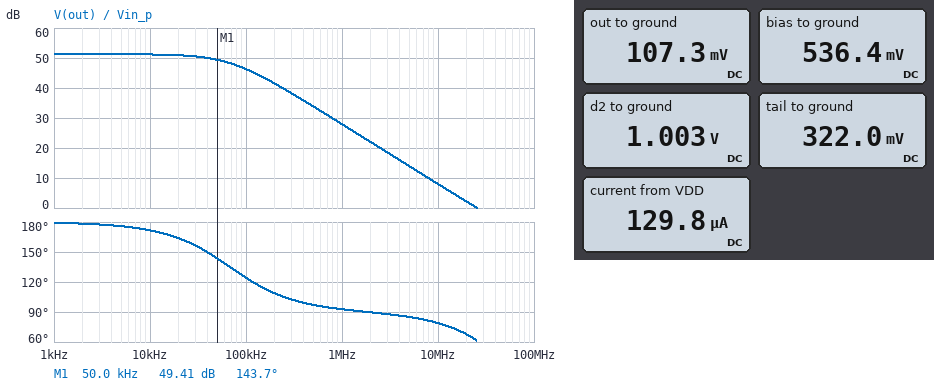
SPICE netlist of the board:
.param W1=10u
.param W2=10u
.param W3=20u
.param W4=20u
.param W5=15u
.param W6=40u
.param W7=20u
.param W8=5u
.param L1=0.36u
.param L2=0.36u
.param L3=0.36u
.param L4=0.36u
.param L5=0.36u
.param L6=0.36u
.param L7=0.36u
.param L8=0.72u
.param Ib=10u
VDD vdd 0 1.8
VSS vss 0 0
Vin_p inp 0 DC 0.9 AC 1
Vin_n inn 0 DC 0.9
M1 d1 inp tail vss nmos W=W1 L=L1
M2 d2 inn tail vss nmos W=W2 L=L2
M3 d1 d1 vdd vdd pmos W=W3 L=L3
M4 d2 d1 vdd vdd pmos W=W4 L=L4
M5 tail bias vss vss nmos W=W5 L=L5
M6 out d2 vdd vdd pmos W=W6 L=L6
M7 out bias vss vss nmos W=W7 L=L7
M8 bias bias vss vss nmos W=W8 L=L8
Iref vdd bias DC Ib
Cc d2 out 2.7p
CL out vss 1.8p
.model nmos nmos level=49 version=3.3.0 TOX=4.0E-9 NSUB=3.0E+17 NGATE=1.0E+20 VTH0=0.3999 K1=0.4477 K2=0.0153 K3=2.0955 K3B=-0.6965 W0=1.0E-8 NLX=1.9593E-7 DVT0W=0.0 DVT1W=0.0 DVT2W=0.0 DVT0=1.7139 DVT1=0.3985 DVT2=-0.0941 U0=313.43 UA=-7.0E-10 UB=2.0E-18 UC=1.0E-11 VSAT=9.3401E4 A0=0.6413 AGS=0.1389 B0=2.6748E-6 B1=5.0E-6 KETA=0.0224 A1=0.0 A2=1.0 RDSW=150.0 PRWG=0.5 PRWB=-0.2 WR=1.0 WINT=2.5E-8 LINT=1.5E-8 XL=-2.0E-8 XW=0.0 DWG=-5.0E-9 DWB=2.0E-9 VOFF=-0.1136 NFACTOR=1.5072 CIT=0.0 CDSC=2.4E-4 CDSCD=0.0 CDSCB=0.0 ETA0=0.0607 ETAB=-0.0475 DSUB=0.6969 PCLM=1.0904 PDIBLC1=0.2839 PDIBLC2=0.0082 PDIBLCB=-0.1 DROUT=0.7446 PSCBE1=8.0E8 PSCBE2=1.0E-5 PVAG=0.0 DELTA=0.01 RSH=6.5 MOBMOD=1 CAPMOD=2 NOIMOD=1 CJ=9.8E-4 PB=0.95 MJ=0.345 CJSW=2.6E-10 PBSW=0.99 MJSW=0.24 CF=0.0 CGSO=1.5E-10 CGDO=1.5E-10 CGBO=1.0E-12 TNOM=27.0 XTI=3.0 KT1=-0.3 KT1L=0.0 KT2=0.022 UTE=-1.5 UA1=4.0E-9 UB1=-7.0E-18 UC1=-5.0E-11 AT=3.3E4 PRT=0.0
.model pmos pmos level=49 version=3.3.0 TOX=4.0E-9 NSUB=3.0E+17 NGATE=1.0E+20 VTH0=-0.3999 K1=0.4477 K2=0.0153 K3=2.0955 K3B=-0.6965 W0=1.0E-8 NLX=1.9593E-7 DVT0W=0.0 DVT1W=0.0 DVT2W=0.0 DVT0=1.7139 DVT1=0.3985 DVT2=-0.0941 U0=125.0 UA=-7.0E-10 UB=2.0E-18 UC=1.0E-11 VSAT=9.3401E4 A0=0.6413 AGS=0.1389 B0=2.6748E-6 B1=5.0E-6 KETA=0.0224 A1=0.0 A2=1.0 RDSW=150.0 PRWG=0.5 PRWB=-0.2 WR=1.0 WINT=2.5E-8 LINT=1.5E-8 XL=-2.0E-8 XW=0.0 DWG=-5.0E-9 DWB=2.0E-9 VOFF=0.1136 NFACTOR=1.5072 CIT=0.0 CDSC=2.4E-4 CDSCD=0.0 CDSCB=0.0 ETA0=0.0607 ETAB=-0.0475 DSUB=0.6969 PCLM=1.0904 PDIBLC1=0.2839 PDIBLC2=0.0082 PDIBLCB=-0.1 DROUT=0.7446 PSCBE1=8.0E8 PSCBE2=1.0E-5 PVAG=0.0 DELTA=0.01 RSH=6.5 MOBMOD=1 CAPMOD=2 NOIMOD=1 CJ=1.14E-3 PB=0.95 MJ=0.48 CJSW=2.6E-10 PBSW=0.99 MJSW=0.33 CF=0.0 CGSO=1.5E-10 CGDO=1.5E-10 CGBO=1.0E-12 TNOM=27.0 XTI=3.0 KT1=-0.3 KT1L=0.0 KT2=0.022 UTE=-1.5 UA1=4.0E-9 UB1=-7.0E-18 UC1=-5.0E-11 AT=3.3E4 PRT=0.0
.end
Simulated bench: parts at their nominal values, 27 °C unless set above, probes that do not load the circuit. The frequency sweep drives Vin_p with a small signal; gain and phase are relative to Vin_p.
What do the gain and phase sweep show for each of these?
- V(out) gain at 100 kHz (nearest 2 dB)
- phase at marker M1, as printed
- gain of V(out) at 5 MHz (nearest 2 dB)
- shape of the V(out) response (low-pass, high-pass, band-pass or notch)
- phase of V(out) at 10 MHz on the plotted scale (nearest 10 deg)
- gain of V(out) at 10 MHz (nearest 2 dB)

46 dB
143.7 deg
14 dB
low-pass
80 deg
8 dB
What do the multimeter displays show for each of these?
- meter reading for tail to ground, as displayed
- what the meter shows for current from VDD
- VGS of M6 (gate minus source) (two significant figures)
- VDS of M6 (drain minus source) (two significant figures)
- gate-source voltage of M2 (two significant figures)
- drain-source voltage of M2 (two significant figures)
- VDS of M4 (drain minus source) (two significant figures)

322.0 mV
129.8 µA
-800 mV
-1.7 V
580 mV
680 mV
-800 mV
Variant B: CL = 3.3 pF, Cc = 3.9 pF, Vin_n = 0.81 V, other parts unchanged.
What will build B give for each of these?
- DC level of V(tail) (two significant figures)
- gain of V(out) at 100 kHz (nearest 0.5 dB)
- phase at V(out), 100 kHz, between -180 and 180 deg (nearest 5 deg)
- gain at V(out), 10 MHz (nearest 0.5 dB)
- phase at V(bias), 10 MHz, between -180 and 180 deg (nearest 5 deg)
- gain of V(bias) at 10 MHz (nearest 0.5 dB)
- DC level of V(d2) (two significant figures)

300 mV
-62.0 dB
90 deg
-24.0 dB
110 deg
-60.0 dB
1.8 V
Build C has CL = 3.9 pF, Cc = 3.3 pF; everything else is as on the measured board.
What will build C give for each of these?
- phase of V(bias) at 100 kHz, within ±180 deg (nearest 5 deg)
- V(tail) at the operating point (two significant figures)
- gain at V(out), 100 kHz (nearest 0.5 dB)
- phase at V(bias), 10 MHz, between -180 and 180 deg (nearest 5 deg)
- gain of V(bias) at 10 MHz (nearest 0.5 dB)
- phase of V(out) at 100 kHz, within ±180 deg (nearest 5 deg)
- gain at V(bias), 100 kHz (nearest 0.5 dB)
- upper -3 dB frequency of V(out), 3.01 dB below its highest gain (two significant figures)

-150 deg
320 mV
45.0 dB
155 deg
-49.5 dB
120 deg
-51.0 dB
56 kHz
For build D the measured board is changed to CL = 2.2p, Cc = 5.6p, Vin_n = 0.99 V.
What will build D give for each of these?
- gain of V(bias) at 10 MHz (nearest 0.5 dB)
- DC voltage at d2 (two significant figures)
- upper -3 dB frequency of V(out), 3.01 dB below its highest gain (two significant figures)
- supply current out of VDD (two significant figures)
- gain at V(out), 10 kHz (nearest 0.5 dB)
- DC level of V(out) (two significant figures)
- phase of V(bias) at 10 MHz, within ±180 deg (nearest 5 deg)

-64.0 dB
360 mV
590 MHz
160 µA
-43.0 dB
1.8 V
70 deg
